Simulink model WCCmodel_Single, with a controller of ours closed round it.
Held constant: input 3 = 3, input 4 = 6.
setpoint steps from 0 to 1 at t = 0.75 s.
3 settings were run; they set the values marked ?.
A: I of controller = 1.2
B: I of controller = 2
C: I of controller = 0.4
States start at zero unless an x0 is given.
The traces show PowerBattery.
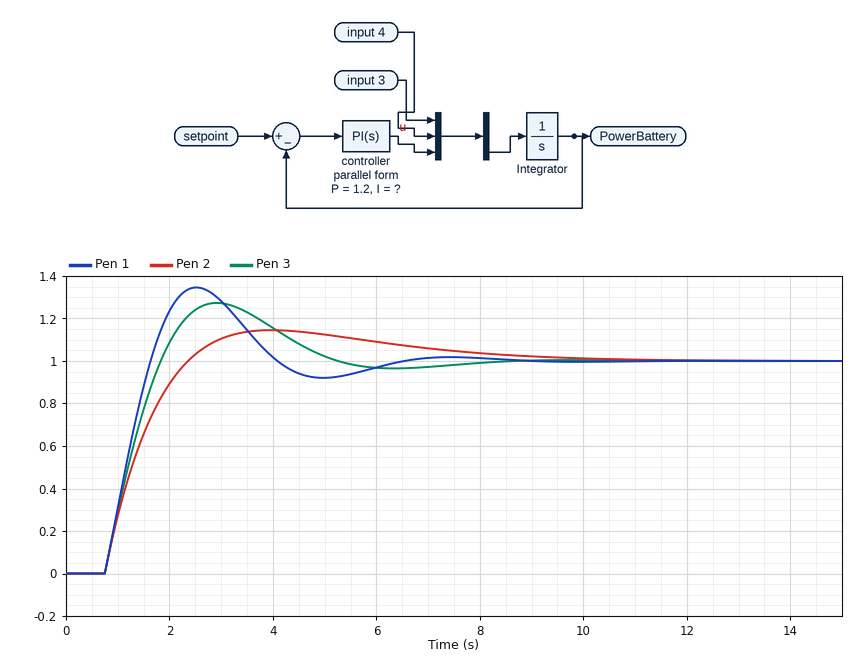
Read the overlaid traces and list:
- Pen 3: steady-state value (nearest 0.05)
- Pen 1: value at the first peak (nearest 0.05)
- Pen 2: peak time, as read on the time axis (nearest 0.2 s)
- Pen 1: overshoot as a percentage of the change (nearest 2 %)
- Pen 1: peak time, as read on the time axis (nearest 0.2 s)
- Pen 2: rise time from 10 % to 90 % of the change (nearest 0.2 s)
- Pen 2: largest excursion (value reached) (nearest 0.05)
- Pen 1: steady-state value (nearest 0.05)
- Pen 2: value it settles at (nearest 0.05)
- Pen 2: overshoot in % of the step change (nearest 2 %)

1.00
1.35
4.0 s
34 %
2.6 s
1.2 s
1.15
1.00
1.00
14 %
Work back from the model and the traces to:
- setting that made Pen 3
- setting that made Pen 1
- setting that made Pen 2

A
B
C
